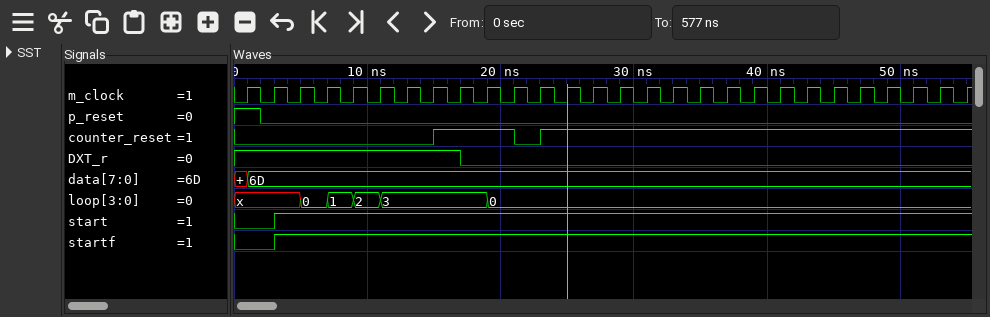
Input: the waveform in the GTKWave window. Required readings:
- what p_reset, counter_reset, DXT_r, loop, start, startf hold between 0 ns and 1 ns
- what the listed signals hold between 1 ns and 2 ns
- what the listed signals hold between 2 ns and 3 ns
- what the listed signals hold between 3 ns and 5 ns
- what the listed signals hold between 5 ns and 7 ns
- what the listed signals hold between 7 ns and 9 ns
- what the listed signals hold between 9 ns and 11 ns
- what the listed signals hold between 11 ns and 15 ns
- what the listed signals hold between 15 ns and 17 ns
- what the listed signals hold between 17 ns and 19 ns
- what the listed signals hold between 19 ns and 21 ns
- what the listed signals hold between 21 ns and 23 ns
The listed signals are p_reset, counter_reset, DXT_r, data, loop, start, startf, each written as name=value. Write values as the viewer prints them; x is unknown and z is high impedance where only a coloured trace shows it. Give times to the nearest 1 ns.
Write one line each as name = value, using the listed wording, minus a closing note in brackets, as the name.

what p_reset, counter_reset, DXT_r, loop, start, startf hold between 0 ns and 1 ns = p_reset=1, counter_reset=0, DXT_r=1, loop=x, start=0, startf=0
what the listed signals hold between 1 ns and 2 ns = p_reset=1, counter_reset=0, DXT_r=1, data=6D, loop=x, start=0, startf=0
what the listed signals hold between 2 ns and 3 ns = p_reset=0, counter_reset=0, DXT_r=1, data=6D, loop=x, start=0, startf=0
what the listed signals hold between 3 ns and 5 ns = p_reset=0, counter_reset=0, DXT_r=1, data=6D, loop=x, start=1, startf=1
what the listed signals hold between 5 ns and 7 ns = p_reset=0, counter_reset=0, DXT_r=1, data=6D, loop=0, start=1, startf=1
what the listed signals hold between 7 ns and 9 ns = p_reset=0, counter_reset=0, DXT_r=1, data=6D, loop=1, start=1, startf=1
what the listed signals hold between 9 ns and 11 ns = p_reset=0, counter_reset=0, DXT_r=1, data=6D, loop=2, start=1, startf=1
what the listed signals hold between 11 ns and 15 ns = p_reset=0, counter_reset=0, DXT_r=1, data=6D, loop=3, start=1, startf=1
what the listed signals hold between 15 ns and 17 ns = p_reset=0, counter_reset=1, DXT_r=1, data=6D, loop=3, start=1, startf=1
what the listed signals hold between 17 ns and 19 ns = p_reset=0, counter_reset=1, DXT_r=0, data=6D, loop=3, start=1, startf=1
what the listed signals hold between 19 ns and 21 ns = p_reset=0, counter_reset=1, DXT_r=0, data=6D, loop=0, start=1, startf=1
what the listed signals hold between 21 ns and 23 ns = p_reset=0, counter_reset=0, DXT_r=0, data=6D, loop=0, start=1, startf=1
